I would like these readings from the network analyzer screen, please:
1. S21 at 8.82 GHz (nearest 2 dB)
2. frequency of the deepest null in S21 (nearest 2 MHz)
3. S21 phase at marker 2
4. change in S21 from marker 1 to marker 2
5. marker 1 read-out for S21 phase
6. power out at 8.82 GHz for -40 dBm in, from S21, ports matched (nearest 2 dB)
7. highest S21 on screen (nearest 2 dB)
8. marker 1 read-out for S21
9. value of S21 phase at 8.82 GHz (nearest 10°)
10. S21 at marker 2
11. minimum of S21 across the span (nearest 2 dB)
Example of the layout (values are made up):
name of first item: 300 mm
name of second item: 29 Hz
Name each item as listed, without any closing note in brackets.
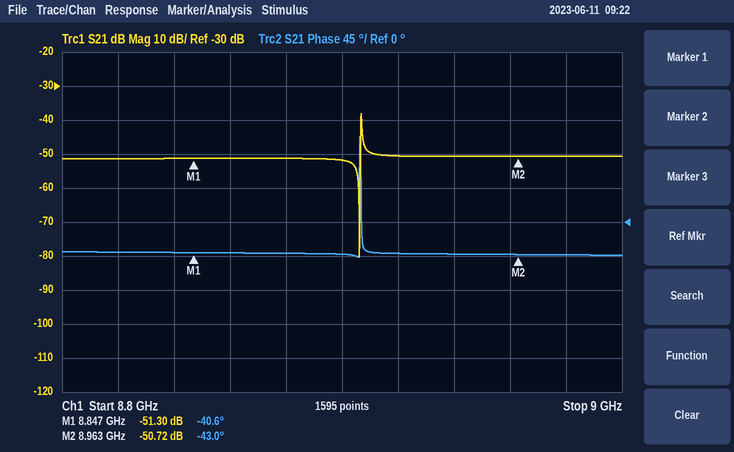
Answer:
S21 at 8.82 GHz: -52 dB
frequency of the deepest null in S21: 8.906 GHz
S21 phase at marker 2: -43.0°
change in S21 from marker 1 to marker 2: 0.58 dB
marker 1 read-out for S21 phase: -40.6°
power out at 8.82 GHz for -40 dBm in, from S21, ports matched: -92 dBm
highest S21 on screen: -38 dB
marker 1 read-out for S21: -51.30 dB
value of S21 phase at 8.82 GHz: -40°
S21 at marker 2: -50.72 dB
minimum of S21 across the span: -80 dB
